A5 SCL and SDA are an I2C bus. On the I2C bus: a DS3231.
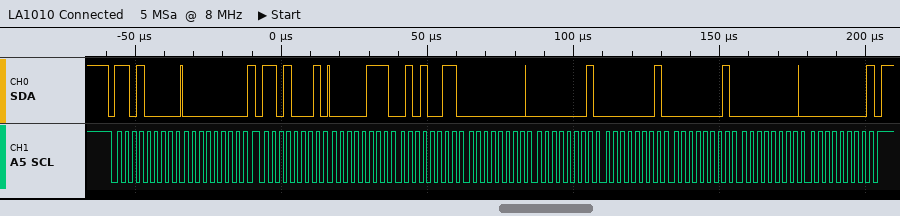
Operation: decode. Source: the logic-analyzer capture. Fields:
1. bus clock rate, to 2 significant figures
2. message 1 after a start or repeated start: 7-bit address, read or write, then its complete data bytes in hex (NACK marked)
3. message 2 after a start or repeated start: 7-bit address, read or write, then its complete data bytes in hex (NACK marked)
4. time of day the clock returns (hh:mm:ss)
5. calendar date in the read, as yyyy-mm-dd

400 kHz
0x68 write: 00
0x68 read: 07 53 00 01 01 01 00 00 NACK
00:53:07
2000-01-01
